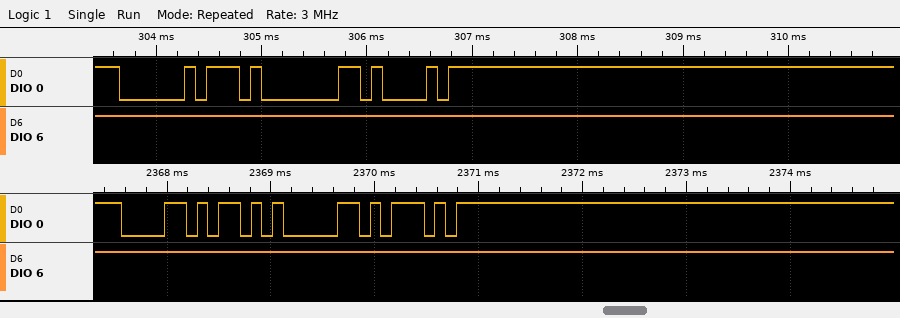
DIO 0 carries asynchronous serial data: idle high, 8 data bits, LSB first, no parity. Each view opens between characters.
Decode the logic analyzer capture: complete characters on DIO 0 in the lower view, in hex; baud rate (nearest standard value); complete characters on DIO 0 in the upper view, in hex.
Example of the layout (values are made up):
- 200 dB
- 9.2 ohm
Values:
- 58, 05, 5D
- 9600 baud
- A0, 01, A1
